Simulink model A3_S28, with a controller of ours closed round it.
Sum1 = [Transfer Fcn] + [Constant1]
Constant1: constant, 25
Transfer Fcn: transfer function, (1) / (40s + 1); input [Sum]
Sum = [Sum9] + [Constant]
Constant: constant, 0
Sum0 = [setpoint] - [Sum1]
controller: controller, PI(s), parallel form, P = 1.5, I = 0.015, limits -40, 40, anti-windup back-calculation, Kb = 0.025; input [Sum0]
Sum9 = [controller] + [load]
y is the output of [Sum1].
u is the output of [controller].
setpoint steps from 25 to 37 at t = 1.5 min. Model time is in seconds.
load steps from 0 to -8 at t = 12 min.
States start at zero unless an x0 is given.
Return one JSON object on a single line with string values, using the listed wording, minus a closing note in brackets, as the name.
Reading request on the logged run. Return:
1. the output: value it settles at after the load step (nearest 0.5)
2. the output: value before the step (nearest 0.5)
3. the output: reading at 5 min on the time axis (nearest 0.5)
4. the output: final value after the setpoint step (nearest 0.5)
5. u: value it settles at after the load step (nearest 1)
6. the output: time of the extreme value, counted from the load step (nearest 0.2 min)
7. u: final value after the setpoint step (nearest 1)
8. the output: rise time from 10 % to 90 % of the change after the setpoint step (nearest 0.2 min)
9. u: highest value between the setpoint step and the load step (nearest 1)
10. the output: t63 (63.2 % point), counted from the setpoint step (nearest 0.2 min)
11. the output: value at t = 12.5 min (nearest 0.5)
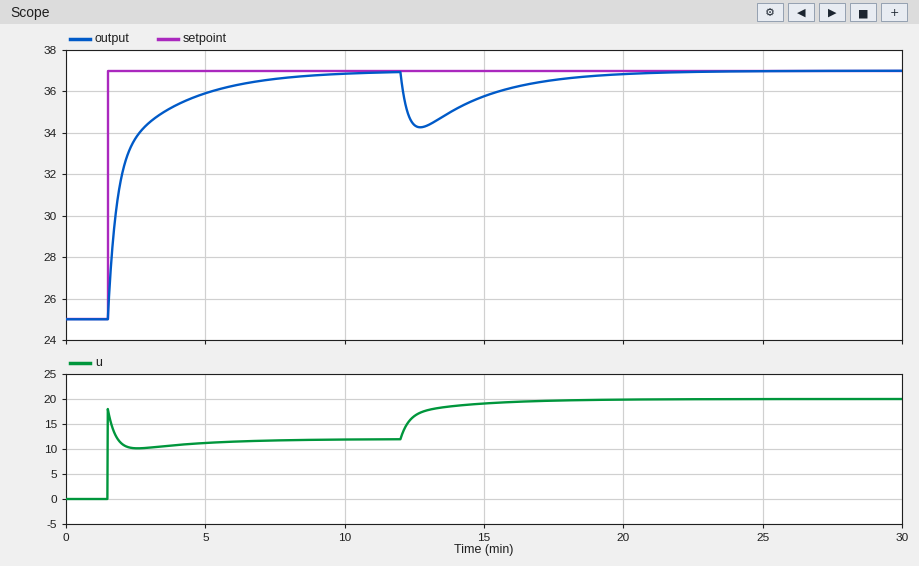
{"the output: value it settles at after the load step": "37.0", "the output: value before the step": "25.0", "the output: reading at 5 min on the time axis": "36.0", "the output: final value after the setpoint step": "37.0", "u: value it settles at after the load step": "20", "the output: time of the extreme value, counted from the load step": "0.8 min", "u: final value after the setpoint step": "12", "the output: rise time from 10 % to 90 % of the change after the setpoint step": "3.2 min", "u: highest value between the setpoint step and the load step": "18", "the output: t63 (63.2 % point), counted from the setpoint step": "0.6 min", "the output: value at t = 12.5 min": "34.5"}
